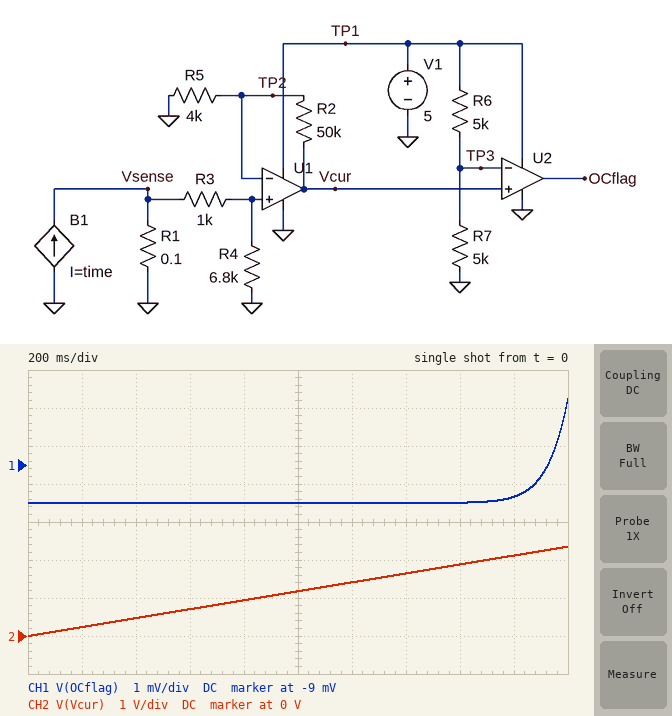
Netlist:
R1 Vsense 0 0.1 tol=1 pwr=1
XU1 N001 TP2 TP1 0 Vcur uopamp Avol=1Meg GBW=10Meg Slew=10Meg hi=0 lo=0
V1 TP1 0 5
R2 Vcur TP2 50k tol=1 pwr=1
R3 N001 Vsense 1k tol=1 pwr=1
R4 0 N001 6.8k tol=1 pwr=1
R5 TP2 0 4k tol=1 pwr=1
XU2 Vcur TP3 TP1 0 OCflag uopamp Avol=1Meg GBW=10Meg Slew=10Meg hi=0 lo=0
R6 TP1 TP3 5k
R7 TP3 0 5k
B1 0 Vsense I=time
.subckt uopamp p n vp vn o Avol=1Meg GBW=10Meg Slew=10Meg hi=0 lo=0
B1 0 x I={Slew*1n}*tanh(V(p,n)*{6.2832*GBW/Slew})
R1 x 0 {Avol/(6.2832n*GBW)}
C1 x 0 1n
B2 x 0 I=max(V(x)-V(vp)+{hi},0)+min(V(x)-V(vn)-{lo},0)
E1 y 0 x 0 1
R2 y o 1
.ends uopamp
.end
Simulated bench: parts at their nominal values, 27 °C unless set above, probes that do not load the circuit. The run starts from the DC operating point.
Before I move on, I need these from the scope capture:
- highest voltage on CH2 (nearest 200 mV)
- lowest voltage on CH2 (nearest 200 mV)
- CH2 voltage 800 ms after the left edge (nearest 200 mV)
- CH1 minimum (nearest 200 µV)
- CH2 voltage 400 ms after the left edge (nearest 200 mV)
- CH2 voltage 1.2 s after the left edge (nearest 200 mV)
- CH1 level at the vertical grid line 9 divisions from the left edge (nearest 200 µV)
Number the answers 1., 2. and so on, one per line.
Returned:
1. 2.4 V
2. 0 V
3. 1.0 V
4. -10.0 mV
5. 400 mV
6. 1.4 V
7. -9.8 mV
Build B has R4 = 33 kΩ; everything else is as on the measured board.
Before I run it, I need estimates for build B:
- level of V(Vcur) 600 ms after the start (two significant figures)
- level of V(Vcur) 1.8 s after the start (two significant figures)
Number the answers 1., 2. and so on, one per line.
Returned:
1. 790 mV
2. 2.4 V
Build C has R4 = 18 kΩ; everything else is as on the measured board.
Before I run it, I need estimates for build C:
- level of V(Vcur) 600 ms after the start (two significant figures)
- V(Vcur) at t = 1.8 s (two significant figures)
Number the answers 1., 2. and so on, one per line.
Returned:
1. 770 mV
2. 2.3 V
